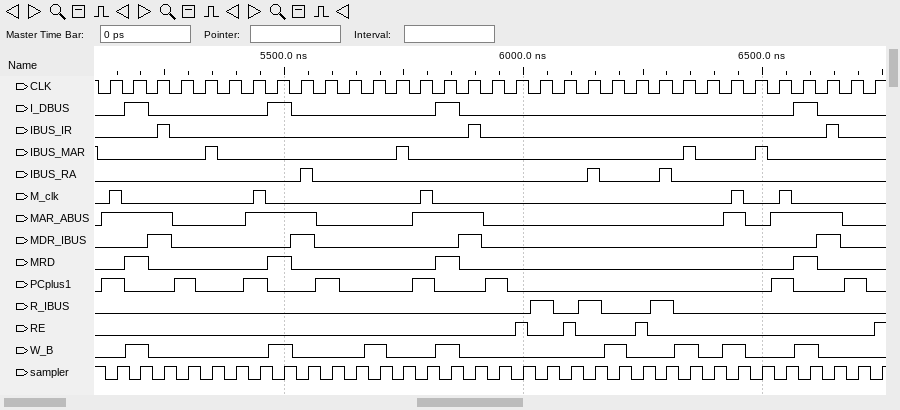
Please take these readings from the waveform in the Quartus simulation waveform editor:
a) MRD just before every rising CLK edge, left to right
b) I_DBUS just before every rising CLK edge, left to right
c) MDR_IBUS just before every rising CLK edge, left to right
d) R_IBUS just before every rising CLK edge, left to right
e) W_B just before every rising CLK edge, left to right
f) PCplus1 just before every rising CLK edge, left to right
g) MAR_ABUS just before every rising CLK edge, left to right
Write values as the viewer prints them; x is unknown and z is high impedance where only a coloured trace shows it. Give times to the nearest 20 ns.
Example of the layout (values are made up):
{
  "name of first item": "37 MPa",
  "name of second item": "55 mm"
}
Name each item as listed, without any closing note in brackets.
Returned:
{
  "MRD just before every rising CLK edge, left to right": "0 1 0 0 0 0 0 1 0 0 0 0 0 0 1 0 0 0 0 0 0 0 0 0 0 0 0 0 0 1 0 0 0",
  "I_DBUS just before every rising CLK edge, left to right": "0 1 0 0 0 0 0 1 0 0 0 0 0 0 1 0 0 0 0 0 0 0 0 0 0 0 0 0 0 1 0 0 0",
  "MDR_IBUS just before every rising CLK edge, left to right": "0 0 1 0 0 0 0 0 1 0 0 0 0 0 0 1 0 0 0 0 0 0 0 0 0 0 0 0 0 0 1 0 0",
  "R_IBUS just before every rising CLK edge, left to right": "0 0 0 0 0 0 0 0 0 0 0 0 0 0 0 0 0 0 1 0 1 0 0 1 0 0 0 0 0 0 0 0 0",
  "W_B just before every rising CLK edge, left to right": "0 1 0 0 0 0 0 1 0 0 0 1 0 0 1 0 0 0 0 0 0 1 0 0 1 0 1 0 0 1 0 0 0",
  "PCplus1 just before every rising CLK edge, left to right": "1 0 0 1 0 0 1 0 0 1 0 0 0 1 0 0 1 0 0 0 0 0 0 0 0 0 0 0 1 0 0 1 0",
  "MAR_ABUS just before every rising CLK edge, left to right": "1 1 1 0 0 0 1 1 1 0 0 0 0 1 1 1 0 0 0 0 0 0 0 0 0 0 1 0 1 1 1 0 0"
}
